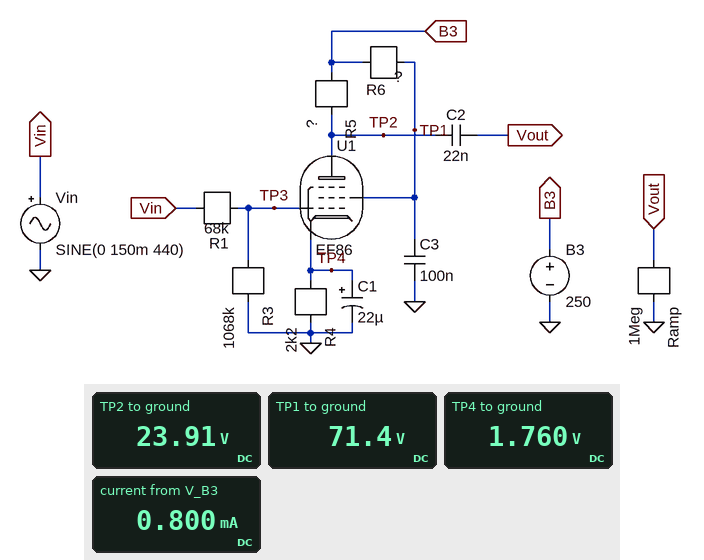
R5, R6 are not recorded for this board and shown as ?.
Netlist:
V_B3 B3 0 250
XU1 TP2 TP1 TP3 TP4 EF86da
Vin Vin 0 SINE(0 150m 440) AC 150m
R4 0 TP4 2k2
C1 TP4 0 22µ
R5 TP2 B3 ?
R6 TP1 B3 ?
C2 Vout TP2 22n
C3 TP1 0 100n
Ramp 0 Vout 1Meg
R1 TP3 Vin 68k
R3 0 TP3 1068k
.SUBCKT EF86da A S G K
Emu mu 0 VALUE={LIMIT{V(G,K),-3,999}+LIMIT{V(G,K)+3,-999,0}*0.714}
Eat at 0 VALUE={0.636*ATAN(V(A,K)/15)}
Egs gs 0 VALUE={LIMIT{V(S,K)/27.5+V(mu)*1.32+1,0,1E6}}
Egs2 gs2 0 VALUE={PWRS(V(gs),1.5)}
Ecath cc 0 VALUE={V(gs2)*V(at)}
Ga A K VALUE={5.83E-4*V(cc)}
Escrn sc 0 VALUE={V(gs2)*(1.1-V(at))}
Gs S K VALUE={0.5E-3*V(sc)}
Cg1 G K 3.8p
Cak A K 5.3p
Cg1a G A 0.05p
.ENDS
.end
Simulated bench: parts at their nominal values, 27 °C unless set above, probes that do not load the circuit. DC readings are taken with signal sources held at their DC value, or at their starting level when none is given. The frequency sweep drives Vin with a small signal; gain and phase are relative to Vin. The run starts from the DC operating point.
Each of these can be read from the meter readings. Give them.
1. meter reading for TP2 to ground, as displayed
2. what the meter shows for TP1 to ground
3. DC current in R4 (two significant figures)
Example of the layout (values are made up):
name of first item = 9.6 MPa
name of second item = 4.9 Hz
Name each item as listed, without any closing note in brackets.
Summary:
meter reading for TP2 to ground, as displayed = 23.91 V
what the meter shows for TP1 to ground = 71.4 V
DC current in R4 = 800 µA
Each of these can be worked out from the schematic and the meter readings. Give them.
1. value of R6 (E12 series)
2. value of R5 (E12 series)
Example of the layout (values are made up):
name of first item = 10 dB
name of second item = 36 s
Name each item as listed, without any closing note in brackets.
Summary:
value of R6 = 560 kΩ
value of R5 = 470 kΩ
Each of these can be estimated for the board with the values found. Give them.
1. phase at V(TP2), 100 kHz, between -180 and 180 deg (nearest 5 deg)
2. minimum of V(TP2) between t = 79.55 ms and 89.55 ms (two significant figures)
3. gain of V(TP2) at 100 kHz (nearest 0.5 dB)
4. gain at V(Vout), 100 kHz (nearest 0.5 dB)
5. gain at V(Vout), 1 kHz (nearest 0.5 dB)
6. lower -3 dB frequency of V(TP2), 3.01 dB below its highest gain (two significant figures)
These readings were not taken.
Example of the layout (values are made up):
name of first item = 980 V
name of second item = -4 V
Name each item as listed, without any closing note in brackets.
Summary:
phase at V(TP2), 100 kHz, between -180 and 180 deg = 150 deg
minimum of V(TP2) between t = 79.55 ms and 89.55 ms = 18 V
gain of V(TP2) at 100 kHz = 34.0 dB
gain at V(Vout), 100 kHz = 34.0 dB
gain at V(Vout), 1 kHz = 35.0 dB
lower -3 dB frequency of V(TP2), 3.01 dB below its highest gain = 57 Hz
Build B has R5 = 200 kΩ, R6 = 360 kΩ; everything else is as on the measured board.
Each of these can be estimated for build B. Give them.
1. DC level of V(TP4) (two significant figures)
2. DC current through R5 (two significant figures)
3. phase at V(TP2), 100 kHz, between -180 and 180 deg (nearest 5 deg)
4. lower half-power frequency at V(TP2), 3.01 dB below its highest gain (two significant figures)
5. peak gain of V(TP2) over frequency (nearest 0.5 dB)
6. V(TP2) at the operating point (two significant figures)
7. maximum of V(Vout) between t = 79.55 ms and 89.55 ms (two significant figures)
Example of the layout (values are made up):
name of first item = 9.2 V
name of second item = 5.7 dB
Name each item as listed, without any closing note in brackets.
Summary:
DC level of V(TP4) = 3.0 V
DC current through R5 = 1.0 mA
phase at V(TP2), 100 kHz, between -180 and 180 deg = 145 deg
lower half-power frequency at V(TP2), 3.01 dB below its highest gain = 53 Hz
peak gain of V(TP2) over frequency = 40.0 dB
V(TP2) at the operating point = 48 V
maximum of V(Vout) between t = 79.55 ms and 89.55 ms = 14 V
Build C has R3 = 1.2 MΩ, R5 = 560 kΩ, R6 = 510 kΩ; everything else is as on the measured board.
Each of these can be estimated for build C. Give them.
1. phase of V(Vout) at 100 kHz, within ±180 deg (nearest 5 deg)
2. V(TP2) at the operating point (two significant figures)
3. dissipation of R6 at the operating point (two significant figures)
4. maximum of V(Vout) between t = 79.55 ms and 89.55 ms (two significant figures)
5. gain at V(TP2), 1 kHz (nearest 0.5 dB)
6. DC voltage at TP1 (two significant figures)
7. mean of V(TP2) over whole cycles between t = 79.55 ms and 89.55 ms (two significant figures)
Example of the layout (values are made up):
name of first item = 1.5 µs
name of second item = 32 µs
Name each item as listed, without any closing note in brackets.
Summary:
phase of V(Vout) at 100 kHz, within ±180 deg = 155 deg
V(TP2) at the operating point = 19 V
dissipation of R6 at the operating point = 65 mW
maximum of V(Vout) between t = 79.55 ms and 89.55 ms = 7.8 V
gain at V(TP2), 1 kHz = 32.0 dB
DC voltage at TP1 = 68 V
mean of V(TP2) over whole cycles between t = 79.55 ms and 89.55 ms = 20 V
